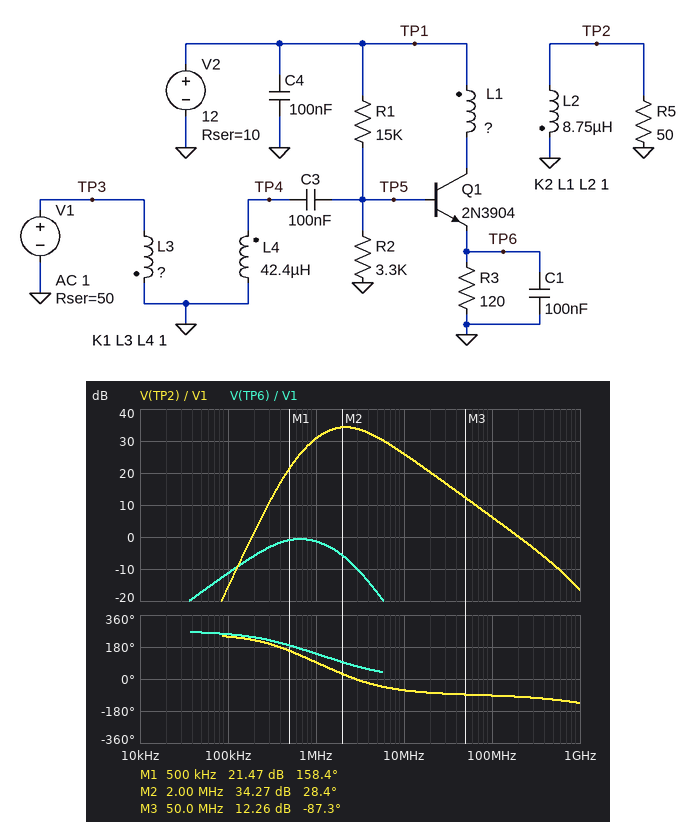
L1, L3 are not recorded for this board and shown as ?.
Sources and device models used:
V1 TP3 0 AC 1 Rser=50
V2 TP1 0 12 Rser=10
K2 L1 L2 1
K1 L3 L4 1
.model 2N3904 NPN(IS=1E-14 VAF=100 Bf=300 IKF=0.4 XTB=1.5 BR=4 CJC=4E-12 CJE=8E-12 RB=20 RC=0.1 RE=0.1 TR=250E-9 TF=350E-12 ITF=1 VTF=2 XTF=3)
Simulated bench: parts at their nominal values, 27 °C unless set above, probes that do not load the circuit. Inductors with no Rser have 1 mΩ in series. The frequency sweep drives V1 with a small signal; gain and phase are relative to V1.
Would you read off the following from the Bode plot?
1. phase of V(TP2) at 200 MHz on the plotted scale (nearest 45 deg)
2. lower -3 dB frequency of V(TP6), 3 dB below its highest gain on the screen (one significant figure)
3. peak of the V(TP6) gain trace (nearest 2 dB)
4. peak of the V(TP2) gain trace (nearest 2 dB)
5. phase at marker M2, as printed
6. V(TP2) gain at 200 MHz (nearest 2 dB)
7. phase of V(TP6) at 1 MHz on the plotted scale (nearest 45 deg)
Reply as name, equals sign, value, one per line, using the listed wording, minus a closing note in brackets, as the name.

phase of V(TP2) at 200 MHz on the plotted scale = -90 deg
lower -3 dB frequency of V(TP6), 3 dB below its highest gain on the screen = 300 kHz
peak of the V(TP6) gain trace = 0 dB
peak of the V(TP2) gain trace = 34 dB
phase at marker M2, as printed = 28.4 deg
V(TP2) gain at 200 MHz = 0 dB
phase of V(TP6) at 1 MHz on the plotted scale = 135 deg
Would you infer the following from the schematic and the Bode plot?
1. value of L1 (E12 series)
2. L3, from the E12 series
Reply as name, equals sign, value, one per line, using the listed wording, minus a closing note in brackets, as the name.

value of L1 = 27 µH
L3, from the E12 series = 12 µH
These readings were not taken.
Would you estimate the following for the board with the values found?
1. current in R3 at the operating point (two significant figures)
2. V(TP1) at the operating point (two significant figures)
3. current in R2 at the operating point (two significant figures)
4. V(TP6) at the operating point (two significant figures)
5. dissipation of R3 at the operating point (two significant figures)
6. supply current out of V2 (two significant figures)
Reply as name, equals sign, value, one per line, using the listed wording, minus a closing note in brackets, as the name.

current in R3 at the operating point = 11 mA
V(TP1) at the operating point = 12 V
current in R2 at the operating point = 620 µA
V(TP6) at the operating point = 1.3 V
dissipation of R3 at the operating point = 15 mW
supply current out of V2 = 12 mA
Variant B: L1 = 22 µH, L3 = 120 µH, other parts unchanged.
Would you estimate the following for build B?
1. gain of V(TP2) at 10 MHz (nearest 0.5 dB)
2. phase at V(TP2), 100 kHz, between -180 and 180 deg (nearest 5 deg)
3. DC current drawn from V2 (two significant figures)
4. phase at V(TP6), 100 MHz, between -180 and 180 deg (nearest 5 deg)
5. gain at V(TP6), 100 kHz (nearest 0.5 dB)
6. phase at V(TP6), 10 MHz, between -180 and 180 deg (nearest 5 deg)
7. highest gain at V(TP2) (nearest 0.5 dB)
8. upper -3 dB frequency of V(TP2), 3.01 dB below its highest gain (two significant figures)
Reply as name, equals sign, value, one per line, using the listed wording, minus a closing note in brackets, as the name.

gain of V(TP2) at 10 MHz = 24.0 dB
phase at V(TP2), 100 kHz, between -180 and 180 deg = -170 deg
DC current drawn from V2 = 12 mA
phase at V(TP6), 100 MHz, between -180 and 180 deg = 25 deg
gain at V(TP6), 100 kHz = -6.5 dB
phase at V(TP6), 10 MHz, between -180 and 180 deg = 65 deg
highest gain at V(TP2) = 25.0 dB
upper -3 dB frequency of V(TP2), 3.01 dB below its highest gain = 20 MHz
